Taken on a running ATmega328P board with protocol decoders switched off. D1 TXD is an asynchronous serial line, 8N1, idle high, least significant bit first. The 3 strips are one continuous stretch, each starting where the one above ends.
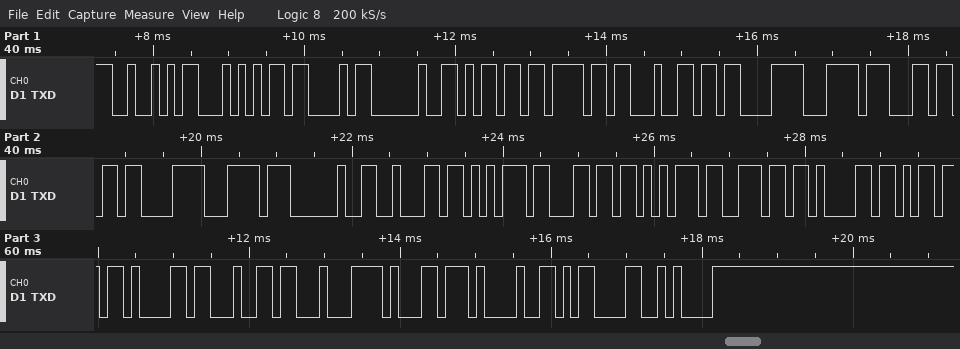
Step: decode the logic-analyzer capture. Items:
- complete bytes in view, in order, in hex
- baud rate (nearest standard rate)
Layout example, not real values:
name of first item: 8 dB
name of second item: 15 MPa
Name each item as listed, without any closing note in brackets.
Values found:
complete bytes in view, in order, in hex: 52 54 43 20 6D 6F 64 C3 BC 6C C3 BC 20 62 75 6C 75 6E 61 6D 61 64 C4 B1 21 0D 0A
baud rate: 9600 baud
